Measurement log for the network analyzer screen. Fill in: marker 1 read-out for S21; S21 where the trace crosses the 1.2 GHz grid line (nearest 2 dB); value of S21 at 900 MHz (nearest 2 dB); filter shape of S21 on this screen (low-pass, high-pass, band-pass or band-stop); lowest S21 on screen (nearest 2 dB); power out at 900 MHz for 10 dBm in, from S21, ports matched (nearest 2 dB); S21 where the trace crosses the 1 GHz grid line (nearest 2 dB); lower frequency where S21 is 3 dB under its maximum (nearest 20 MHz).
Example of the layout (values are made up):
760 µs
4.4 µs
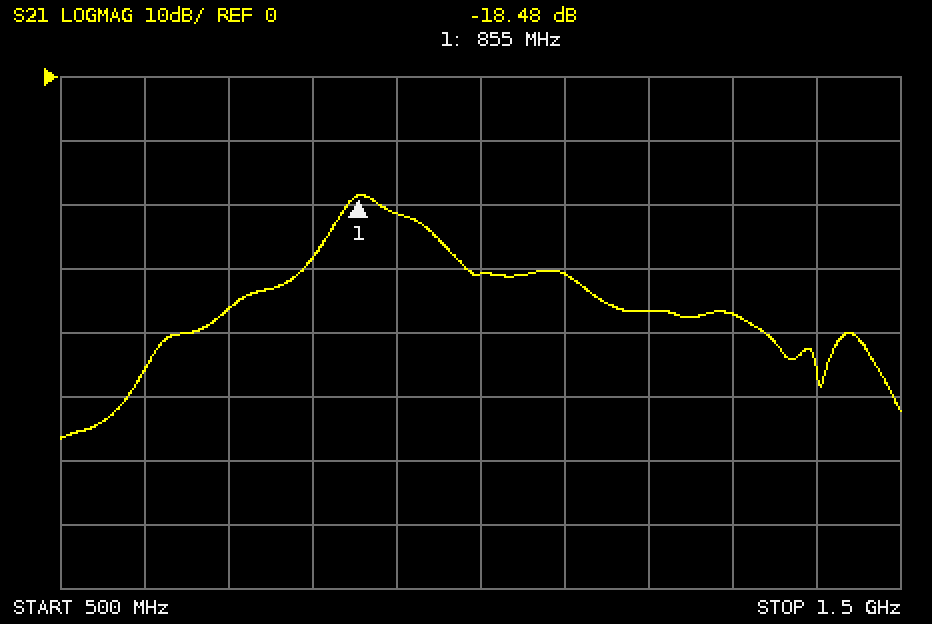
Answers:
-18.48 dB
-36 dB
-22 dB
band-pass
-56 dB
-12 dBm
-30 dB
840 MHz
